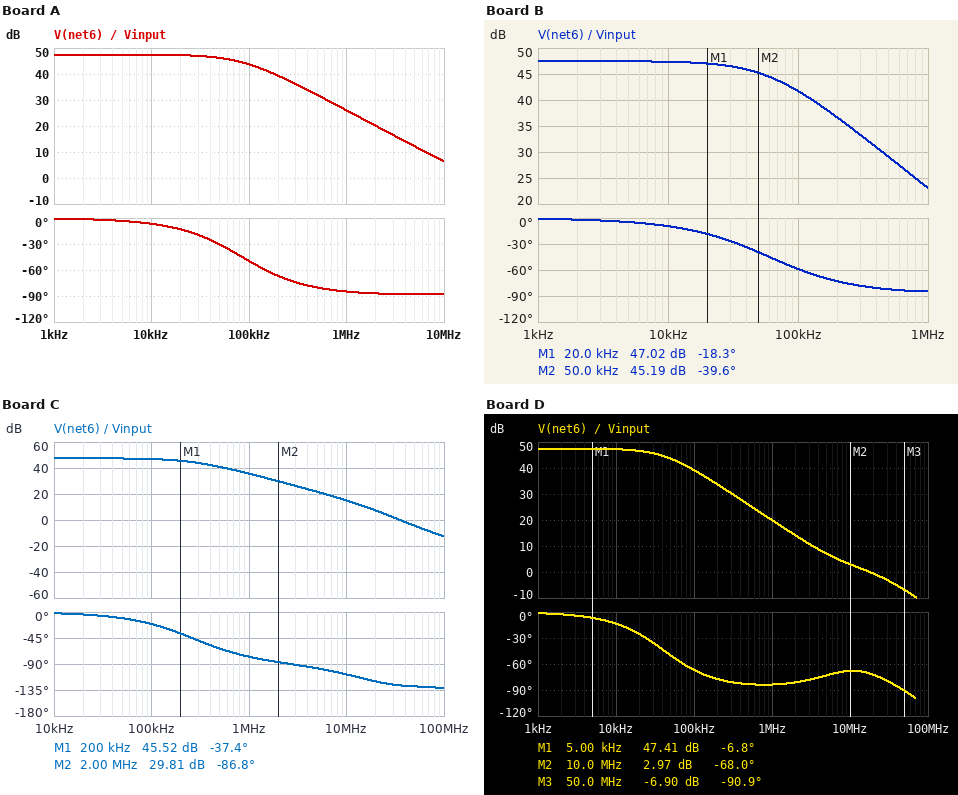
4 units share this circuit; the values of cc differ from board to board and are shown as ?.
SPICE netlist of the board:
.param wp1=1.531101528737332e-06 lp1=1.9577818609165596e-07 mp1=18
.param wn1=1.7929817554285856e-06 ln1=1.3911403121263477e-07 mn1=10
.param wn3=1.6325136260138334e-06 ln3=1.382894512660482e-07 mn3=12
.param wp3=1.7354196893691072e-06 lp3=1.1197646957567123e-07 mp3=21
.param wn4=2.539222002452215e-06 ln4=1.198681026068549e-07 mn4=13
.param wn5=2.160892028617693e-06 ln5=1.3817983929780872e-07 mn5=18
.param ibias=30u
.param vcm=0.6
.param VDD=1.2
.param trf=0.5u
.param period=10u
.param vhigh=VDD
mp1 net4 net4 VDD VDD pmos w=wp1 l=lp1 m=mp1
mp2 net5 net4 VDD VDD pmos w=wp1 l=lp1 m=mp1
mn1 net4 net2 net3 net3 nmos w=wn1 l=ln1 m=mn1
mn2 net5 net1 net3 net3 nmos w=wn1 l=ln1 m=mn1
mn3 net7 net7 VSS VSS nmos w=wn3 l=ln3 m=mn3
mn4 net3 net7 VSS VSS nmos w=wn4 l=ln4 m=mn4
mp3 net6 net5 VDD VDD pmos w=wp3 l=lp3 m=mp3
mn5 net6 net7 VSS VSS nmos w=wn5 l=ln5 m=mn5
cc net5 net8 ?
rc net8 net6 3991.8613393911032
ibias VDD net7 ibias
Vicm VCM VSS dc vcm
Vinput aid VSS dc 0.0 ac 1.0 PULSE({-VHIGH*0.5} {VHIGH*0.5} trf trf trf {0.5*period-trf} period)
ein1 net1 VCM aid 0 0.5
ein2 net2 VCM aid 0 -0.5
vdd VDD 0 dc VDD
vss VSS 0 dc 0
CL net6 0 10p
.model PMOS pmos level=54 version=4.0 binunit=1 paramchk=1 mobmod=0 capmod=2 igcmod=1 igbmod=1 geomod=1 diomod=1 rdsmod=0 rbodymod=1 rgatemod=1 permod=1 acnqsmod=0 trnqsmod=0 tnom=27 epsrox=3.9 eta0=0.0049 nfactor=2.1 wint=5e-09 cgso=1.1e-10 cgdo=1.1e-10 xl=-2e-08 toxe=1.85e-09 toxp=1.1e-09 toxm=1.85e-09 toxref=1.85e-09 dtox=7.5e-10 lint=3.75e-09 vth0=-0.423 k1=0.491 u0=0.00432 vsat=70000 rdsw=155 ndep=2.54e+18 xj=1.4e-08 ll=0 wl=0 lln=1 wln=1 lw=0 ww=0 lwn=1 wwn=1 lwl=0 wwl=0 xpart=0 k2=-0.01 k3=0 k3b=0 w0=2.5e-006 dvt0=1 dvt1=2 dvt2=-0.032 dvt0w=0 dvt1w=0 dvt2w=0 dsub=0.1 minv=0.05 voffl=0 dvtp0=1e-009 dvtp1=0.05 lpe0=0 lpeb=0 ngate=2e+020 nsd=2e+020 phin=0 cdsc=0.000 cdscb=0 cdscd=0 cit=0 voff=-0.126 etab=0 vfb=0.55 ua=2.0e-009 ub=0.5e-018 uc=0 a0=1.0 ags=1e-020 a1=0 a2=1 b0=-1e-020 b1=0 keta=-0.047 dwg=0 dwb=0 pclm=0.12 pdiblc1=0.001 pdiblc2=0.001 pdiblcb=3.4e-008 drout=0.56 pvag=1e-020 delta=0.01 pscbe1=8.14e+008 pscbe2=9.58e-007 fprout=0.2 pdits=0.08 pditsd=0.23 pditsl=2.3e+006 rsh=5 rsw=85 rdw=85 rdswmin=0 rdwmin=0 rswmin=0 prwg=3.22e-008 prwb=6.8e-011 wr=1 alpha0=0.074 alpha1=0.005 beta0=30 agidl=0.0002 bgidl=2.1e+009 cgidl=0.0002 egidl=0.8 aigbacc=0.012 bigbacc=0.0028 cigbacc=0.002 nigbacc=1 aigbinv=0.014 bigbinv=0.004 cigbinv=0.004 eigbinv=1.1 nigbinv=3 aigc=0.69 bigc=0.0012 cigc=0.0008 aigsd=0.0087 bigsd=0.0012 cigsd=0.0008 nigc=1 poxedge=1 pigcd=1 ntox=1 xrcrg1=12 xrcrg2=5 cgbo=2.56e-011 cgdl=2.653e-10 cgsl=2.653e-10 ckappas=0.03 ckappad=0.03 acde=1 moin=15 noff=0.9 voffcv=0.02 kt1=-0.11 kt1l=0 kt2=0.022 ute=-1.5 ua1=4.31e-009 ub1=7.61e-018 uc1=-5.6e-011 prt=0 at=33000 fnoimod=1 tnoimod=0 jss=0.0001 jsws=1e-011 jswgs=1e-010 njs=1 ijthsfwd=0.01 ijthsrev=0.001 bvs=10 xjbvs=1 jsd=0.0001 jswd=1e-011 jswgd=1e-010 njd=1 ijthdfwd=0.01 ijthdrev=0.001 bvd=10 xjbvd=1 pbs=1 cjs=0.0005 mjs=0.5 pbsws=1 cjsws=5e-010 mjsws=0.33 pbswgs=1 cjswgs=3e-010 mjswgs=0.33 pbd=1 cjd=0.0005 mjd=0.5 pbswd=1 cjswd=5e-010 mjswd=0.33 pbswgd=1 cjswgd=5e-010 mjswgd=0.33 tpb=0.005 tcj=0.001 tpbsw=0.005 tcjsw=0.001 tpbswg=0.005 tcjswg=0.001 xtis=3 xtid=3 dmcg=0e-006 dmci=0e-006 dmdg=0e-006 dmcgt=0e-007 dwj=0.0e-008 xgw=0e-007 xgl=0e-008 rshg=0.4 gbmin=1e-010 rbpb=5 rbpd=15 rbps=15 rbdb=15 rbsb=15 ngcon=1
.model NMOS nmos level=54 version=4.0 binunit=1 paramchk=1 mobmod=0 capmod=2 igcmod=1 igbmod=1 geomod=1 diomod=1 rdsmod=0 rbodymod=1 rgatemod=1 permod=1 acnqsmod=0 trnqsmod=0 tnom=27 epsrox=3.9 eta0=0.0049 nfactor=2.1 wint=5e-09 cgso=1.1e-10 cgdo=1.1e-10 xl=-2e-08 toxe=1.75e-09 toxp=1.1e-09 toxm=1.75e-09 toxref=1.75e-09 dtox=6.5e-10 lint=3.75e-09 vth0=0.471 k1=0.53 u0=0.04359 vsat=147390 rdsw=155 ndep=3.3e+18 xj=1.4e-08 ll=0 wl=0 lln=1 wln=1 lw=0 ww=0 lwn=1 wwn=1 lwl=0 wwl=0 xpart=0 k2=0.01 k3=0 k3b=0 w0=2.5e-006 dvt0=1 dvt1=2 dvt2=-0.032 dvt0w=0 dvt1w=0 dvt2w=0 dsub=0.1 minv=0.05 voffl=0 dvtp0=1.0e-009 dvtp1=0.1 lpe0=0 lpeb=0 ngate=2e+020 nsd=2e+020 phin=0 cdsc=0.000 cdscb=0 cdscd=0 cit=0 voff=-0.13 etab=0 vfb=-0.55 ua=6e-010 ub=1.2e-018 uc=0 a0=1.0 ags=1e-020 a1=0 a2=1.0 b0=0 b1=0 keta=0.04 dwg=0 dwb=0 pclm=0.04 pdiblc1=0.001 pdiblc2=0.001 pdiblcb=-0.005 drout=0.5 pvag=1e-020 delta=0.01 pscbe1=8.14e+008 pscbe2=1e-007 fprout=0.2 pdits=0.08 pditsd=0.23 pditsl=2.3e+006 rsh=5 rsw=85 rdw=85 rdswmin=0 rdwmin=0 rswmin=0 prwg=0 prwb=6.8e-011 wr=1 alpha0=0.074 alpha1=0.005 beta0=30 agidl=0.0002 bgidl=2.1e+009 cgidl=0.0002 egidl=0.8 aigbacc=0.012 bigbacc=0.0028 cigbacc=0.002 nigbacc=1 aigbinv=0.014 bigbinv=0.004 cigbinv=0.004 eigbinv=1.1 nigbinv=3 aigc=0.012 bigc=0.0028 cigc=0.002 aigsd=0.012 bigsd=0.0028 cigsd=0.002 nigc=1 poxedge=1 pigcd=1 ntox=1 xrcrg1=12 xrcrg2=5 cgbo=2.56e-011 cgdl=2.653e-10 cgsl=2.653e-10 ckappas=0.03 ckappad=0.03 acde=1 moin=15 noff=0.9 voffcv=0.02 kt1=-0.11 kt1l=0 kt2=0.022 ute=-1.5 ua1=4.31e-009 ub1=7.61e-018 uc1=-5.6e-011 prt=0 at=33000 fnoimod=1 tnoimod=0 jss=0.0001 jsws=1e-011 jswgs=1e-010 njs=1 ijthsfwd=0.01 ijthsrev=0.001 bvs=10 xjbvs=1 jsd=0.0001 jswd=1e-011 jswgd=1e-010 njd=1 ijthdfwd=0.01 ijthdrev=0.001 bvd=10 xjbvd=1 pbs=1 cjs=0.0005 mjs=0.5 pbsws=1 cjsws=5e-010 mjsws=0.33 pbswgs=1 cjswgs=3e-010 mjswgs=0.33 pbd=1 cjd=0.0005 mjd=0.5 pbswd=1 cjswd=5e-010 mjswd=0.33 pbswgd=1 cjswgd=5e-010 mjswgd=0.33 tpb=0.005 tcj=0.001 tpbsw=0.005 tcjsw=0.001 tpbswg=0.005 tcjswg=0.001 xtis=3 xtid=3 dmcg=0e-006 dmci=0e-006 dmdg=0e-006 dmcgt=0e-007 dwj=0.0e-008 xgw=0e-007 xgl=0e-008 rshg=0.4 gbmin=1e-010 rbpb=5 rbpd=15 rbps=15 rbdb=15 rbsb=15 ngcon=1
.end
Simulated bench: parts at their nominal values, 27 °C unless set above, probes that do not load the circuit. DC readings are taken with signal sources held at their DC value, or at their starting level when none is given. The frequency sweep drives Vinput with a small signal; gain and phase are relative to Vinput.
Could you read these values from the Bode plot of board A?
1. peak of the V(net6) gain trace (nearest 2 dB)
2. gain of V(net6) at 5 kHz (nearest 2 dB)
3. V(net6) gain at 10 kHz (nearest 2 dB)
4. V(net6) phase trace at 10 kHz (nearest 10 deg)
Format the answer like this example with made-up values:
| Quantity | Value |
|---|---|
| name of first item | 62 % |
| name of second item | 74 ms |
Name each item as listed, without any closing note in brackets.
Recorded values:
| Quantity | Value |
|---|---|
| peak of the V(net6) gain trace | 48 dB |
| gain of V(net6) at 5 kHz | 48 dB |
| V(net6) gain at 10 kHz | 48 dB |
| V(net6) phase trace at 10 kHz | -10 deg |
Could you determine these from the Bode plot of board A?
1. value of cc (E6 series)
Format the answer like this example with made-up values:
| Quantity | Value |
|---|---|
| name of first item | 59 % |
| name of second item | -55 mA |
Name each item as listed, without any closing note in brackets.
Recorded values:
| Quantity | Value |
|---|---|
| value of cc | 3.3 pF |
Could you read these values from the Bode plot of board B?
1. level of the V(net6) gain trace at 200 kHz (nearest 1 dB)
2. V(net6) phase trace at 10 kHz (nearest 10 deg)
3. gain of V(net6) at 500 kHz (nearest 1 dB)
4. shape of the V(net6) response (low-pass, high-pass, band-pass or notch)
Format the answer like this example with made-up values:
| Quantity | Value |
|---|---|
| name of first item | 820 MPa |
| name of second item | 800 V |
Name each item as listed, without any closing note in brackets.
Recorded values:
| Quantity | Value |
|---|---|
| level of the V(net6) gain trace at 200 kHz | 37 dB |
| V(net6) phase trace at 10 kHz | -10 deg |
| gain of V(net6) at 500 kHz | 29 dB |
| shape of the V(net6) response | low-pass |
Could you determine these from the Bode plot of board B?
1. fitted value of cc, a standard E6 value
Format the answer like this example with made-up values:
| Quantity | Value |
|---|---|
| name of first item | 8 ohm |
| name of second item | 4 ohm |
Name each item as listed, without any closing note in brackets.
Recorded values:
| Quantity | Value |
|---|---|
| fitted value of cc, a standard E6 value | 4.7 pF |
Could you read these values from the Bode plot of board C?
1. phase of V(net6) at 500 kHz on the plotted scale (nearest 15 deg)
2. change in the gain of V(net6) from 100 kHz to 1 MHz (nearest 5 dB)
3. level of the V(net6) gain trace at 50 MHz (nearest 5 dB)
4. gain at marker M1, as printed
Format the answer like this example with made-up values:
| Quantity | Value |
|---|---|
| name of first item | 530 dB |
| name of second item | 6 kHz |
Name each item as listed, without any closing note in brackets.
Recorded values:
| Quantity | Value |
|---|---|
| phase of V(net6) at 500 kHz on the plotted scale | -60 deg |
| change in the gain of V(net6) from 100 kHz to 1 MHz | -10 dB |
| level of the V(net6) gain trace at 50 MHz | -5 dB |
| gain at marker M1, as printed | 45.52 dB |
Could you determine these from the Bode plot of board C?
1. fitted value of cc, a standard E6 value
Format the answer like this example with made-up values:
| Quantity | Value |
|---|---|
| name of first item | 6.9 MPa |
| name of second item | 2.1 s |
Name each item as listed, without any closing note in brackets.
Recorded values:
| Quantity | Value |
|---|---|
| fitted value of cc, a standard E6 value | 1 pF |
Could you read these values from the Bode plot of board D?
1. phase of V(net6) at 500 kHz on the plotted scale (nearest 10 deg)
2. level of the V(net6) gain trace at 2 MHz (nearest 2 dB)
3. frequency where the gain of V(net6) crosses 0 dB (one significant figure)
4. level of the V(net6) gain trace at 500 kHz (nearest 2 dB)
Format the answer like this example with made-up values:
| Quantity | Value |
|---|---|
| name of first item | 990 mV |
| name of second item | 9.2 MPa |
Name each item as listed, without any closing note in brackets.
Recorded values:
| Quantity | Value |
|---|---|
| phase of V(net6) at 500 kHz on the plotted scale | -80 deg |
| level of the V(net6) gain trace at 2 MHz | 14 dB |
| frequency where the gain of V(net6) crosses 0 dB | 20 MHz |
| level of the V(net6) gain trace at 500 kHz | 26 dB |
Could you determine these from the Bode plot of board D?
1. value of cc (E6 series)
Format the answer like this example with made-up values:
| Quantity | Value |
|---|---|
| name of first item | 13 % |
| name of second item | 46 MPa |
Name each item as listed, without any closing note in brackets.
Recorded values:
| Quantity | Value |
|---|---|
| value of cc | 6.8 pF |
